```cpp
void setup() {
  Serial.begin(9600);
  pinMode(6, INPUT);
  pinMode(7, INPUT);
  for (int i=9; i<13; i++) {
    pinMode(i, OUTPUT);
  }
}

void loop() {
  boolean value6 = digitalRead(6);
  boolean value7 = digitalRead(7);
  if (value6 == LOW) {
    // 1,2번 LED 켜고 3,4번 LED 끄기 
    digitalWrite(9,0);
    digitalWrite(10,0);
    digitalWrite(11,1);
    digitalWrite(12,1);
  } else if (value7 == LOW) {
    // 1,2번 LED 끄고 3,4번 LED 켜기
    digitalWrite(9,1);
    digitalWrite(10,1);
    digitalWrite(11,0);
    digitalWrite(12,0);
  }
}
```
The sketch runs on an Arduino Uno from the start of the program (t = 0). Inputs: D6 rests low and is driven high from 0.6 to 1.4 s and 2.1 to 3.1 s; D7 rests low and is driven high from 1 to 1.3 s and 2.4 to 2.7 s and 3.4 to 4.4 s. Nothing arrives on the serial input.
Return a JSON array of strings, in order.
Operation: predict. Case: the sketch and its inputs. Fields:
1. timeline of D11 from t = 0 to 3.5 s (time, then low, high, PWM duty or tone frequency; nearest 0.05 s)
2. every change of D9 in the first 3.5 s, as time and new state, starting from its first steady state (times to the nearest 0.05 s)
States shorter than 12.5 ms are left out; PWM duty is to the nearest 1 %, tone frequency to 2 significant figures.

["0 s high; 0.6 s low; 1.4 s high; 2.1 s low; 3.1 s high", "0 s low; 0.6 s high; 1.4 s low; 2.1 s high; 3.1 s low"]
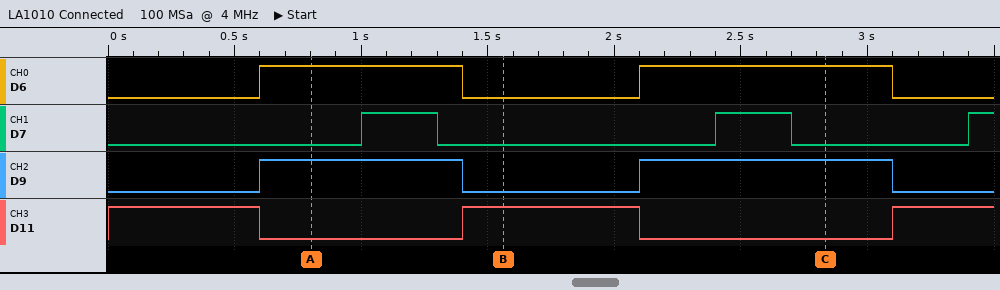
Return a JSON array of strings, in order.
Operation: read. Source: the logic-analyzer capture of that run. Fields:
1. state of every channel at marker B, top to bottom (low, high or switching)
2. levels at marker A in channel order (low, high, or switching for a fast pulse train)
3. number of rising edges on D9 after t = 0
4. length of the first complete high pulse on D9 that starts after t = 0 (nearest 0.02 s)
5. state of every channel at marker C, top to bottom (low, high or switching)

["D6 low, D7 low, D9 low, D11 high", "D6 high, D7 low, D9 high, D11 low", "2", "0.80 s", "D6 high, D7 low, D9 high, D11 low"]
